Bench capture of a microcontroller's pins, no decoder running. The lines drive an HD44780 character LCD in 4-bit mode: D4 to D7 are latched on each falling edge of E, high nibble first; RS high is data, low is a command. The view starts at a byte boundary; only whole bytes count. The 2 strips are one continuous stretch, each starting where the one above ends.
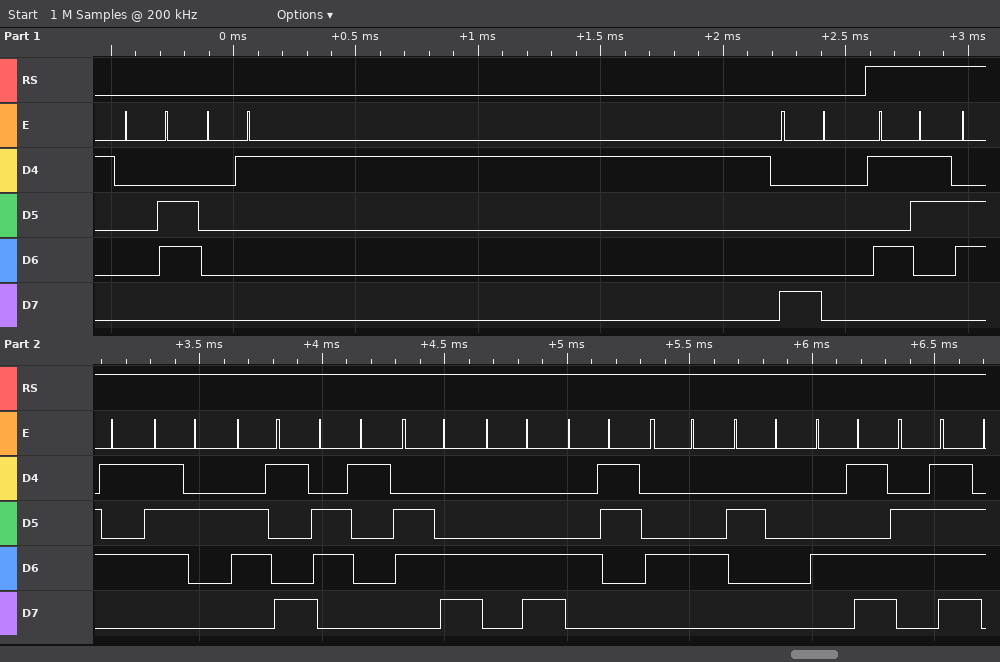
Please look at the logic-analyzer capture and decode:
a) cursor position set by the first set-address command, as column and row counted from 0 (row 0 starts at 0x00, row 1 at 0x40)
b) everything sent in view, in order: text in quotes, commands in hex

column 0, row 0
0x06 0x01 0x80 "SerialLCD Mo"
